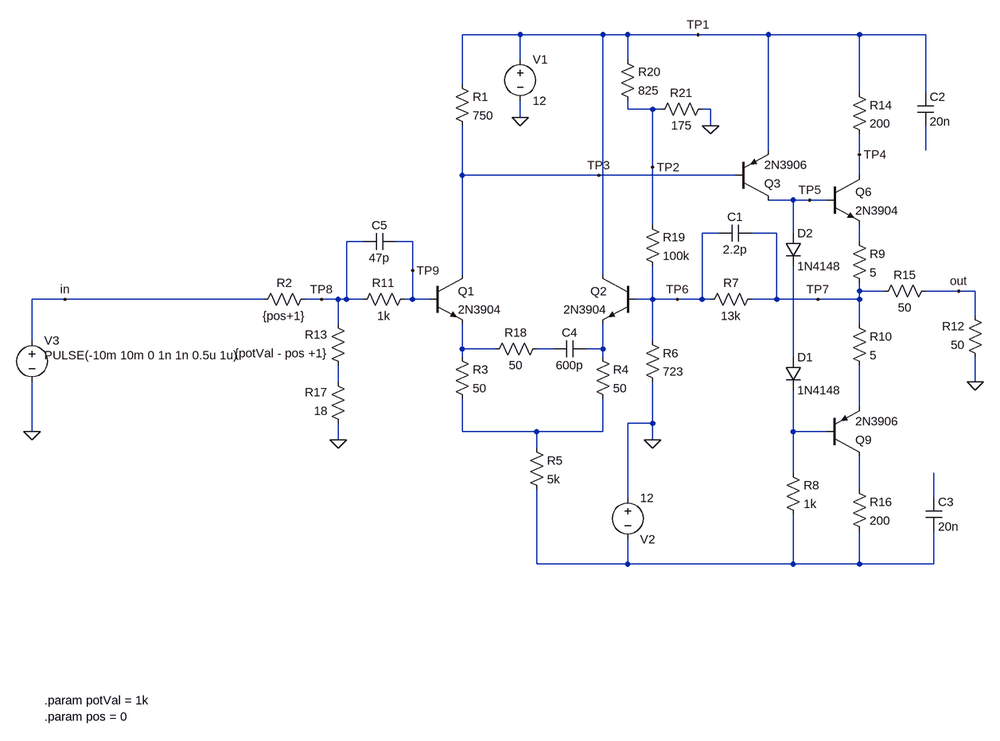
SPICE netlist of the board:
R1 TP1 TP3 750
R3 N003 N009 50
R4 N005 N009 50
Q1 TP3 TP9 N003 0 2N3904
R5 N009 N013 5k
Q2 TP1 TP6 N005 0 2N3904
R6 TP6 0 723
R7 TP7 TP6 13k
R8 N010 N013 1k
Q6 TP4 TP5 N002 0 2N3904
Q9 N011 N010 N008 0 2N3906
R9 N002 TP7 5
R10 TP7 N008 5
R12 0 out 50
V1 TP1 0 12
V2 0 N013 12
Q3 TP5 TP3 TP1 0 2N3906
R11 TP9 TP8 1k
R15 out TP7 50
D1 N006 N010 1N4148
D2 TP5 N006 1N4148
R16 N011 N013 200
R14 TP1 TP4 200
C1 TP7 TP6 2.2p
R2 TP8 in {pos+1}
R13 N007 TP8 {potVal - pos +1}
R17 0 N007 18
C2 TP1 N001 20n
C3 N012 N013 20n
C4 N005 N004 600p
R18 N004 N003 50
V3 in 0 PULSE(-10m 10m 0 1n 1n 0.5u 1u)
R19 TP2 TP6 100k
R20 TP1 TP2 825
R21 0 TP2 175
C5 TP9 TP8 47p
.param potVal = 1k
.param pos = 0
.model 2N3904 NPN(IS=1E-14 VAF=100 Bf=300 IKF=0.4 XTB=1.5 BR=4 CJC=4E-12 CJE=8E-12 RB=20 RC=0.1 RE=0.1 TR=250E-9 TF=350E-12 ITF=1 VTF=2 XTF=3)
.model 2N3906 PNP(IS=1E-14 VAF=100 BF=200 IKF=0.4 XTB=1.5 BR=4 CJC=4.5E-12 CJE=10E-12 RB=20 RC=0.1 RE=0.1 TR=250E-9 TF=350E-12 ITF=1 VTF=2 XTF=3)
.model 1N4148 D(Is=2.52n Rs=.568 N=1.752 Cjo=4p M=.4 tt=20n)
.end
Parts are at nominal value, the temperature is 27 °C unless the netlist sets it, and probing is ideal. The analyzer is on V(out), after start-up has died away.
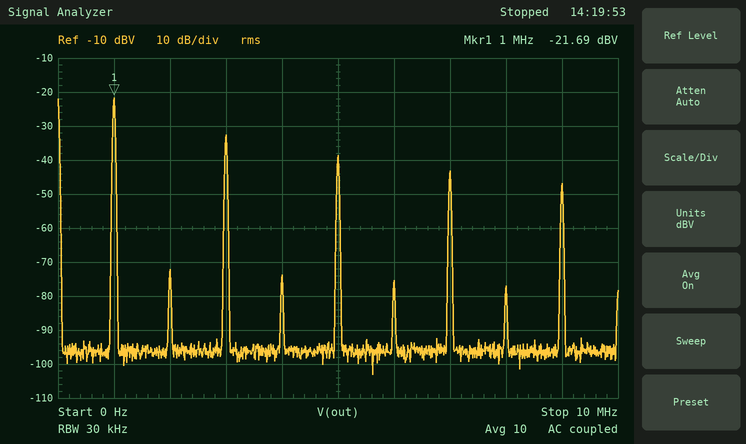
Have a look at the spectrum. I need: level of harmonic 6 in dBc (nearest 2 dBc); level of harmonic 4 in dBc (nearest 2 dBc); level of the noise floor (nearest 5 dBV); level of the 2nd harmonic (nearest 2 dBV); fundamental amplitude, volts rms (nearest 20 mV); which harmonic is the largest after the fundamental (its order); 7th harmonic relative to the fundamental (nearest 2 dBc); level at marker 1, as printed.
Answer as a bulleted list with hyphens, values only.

- -54 dBc
- -52 dBc
- -95 dBV
- -72 dBV
- 80 mV
- 3
- -22 dBc
- -21.69 dBV
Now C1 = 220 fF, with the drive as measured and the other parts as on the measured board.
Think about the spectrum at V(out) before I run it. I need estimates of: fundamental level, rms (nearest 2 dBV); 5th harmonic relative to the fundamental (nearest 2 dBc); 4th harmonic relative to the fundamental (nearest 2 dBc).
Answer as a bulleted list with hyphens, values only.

- -22 dBV
- -14 dBc
- -50 dBc
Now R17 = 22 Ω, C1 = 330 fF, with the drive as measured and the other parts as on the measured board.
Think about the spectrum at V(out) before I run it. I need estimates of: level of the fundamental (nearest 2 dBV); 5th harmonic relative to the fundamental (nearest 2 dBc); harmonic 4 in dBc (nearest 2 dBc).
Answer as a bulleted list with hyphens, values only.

- -22 dBV
- -14 dBc
- -50 dBc
